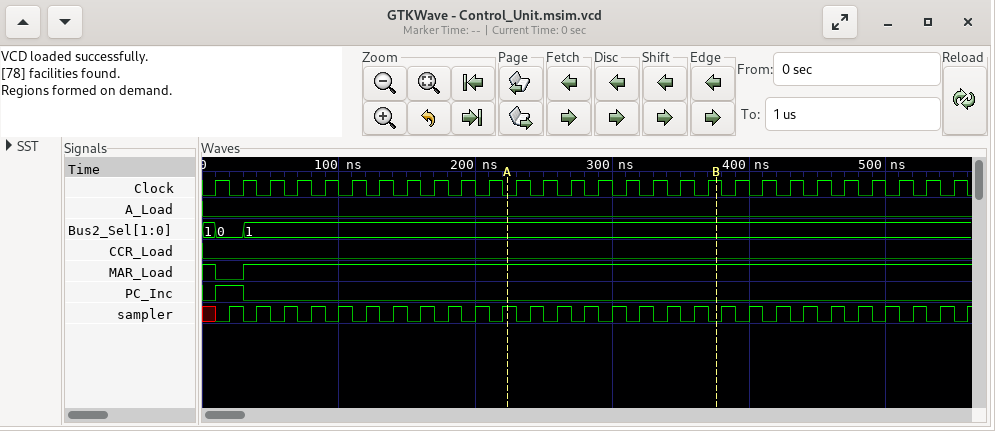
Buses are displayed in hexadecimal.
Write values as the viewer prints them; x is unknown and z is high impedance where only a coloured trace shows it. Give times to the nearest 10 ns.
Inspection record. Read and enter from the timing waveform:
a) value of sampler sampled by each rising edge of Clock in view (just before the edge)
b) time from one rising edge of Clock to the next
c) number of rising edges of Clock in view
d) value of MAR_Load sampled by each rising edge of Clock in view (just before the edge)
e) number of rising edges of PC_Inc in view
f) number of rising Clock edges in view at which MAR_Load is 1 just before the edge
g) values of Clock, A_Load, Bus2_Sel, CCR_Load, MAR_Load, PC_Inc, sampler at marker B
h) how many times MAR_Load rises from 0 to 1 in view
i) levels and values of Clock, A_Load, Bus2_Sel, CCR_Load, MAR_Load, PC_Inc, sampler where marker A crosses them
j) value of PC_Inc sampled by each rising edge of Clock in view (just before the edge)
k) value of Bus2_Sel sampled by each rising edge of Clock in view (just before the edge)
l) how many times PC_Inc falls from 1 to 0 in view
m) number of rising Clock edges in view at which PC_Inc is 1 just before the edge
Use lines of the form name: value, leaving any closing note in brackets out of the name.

value of sampler sampled by each rising edge of Clock in view: x 1 1 1 1 1 1 1 1 1 1 1 1 1 1 1 1 1 1 1 1 1 1 1 1 1 1 1
time from one rising edge of Clock to the next: 20 ns
number of rising edges of Clock in view: 28
value of MAR_Load sampled by each rising edge of Clock in view: 1 0 1 1 1 1 1 1 1 1 1 1 1 1 1 1 1 1 1 1 1 1 1 1 1 1 1 1
number of rising edges of PC_Inc in view: 1
number of rising Clock edges in view at which MAR_Load is 1 just before the edge: 27
values of Clock, A_Load, Bus2_Sel, CCR_Load, MAR_Load, PC_Inc, sampler at marker B: Clock=1, A_Load=0, Bus2_Sel=1, CCR_Load=0, MAR_Load=1, PC_Inc=0, sampler=0
how many times MAR_Load rises from 0 to 1 in view: 1
levels and values of Clock, A_Load, Bus2_Sel, CCR_Load, MAR_Load, PC_Inc, sampler where marker A crosses them: Clock=0, A_Load=0, Bus2_Sel=1, CCR_Load=0, MAR_Load=1, PC_Inc=0, sampler=1
value of PC_Inc sampled by each rising edge of Clock in view: 0 1 0 0 0 0 0 0 0 0 0 0 0 0 0 0 0 0 0 0 0 0 0 0 0 0 0 0
value of Bus2_Sel sampled by each rising edge of Clock in view: 1, 0, 1, 1, 1, 1, 1, 1, 1, 1, 1, 1, 1, 1, 1, 1, 1, 1, 1, 1, 1, 1, 1, 1, 1, 1, 1, 1
how many times PC_Inc falls from 1 to 0 in view: 1
number of rising Clock edges in view at which PC_Inc is 1 just before the edge: 1
